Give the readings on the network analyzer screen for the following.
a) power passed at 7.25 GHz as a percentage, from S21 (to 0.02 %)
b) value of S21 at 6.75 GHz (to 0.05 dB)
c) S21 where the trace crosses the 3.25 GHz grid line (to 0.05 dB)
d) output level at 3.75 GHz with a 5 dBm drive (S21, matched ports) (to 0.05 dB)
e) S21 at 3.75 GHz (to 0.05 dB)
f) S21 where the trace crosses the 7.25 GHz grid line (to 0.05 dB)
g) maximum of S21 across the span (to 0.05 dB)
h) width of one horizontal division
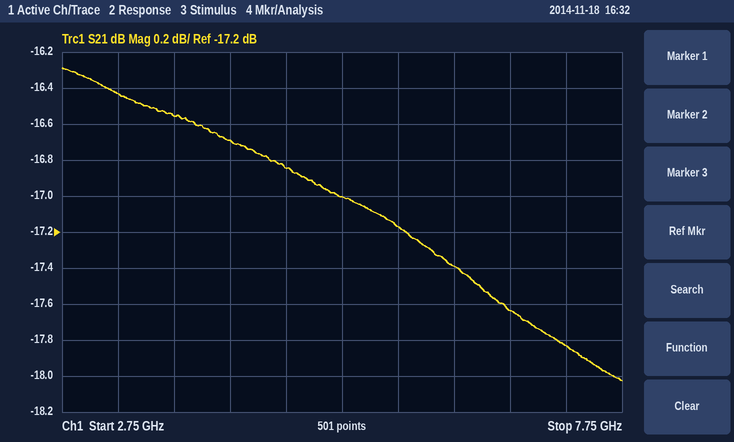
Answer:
1.64 %
-17.65 dB
-16.45 dB
-11.55 dBm
-16.55 dB
-17.85 dB
-16.30 dB
500 MHz
